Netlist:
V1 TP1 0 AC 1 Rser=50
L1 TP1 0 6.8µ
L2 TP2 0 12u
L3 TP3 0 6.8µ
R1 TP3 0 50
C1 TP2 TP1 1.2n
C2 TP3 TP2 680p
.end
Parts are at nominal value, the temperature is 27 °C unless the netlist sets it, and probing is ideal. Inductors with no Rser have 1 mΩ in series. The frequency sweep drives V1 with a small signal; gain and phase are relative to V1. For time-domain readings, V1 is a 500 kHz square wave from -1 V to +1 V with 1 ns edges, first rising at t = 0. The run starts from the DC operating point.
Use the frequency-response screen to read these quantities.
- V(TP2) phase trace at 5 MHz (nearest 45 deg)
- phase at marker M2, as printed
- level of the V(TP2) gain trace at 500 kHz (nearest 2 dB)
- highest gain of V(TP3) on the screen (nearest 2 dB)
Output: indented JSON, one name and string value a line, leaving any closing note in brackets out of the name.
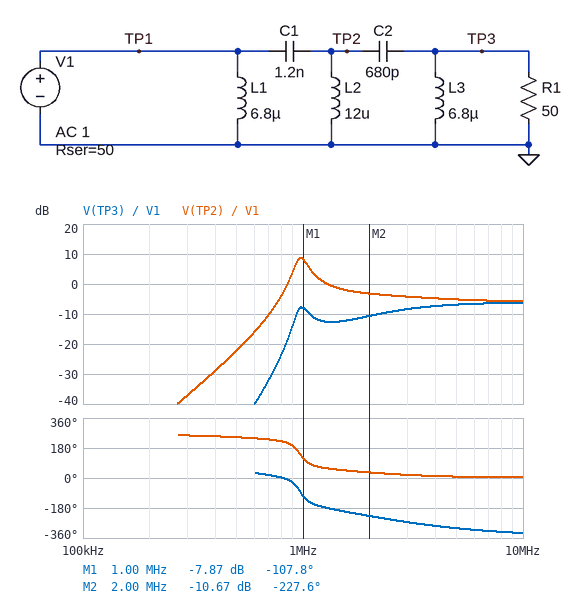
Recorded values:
{
  "V(TP2) phase trace at 5 MHz": "0 deg",
  "phase at marker M2, as printed": "-227.6 deg",
  "level of the V(TP2) gain trace at 500 kHz": "-22 dB",
  "highest gain of V(TP3) on the screen": "-6 dB"
}
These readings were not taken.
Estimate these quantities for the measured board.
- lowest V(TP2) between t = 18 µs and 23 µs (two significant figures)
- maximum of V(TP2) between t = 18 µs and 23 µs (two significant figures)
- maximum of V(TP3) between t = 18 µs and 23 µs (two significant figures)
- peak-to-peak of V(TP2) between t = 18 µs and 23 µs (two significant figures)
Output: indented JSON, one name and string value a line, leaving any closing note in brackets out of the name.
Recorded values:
{
  "lowest V(TP2) between t = 18 µs and 23 µs": "-810 mV",
  "maximum of V(TP2) between t = 18 µs and 23 µs": "810 mV",
  "maximum of V(TP3) between t = 18 µs and 23 µs": "1.0 V",
  "peak-to-peak of V(TP2) between t = 18 µs and 23 µs": "1.6 V"
}
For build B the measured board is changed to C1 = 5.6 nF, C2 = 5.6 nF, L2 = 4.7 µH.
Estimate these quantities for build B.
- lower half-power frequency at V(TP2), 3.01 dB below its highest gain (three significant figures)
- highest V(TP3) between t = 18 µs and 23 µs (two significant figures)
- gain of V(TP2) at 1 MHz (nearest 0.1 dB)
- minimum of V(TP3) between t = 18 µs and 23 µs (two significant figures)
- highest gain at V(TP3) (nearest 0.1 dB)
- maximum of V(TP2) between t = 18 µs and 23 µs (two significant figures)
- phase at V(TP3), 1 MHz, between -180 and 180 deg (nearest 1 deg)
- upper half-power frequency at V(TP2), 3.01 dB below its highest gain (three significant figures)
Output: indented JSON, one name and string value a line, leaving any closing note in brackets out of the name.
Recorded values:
{
  "lower half-power frequency at V(TP2), 3.01 dB below its highest gain": "508 kHz",
  "highest V(TP3) between t = 18 µs and 23 µs": "980 mV",
  "gain of V(TP2) at 1 MHz": "-9.8 dB",
  "minimum of V(TP3) between t = 18 µs and 23 µs": "-980 mV",
  "highest gain at V(TP3)": "-6.0 dB",
  "maximum of V(TP2) between t = 18 µs and 23 µs": "730 mV",
  "phase at V(TP3), 1 MHz, between -180 and 180 deg": "130 deg",
  "upper half-power frequency at V(TP2), 3.01 dB below its highest gain": "620 kHz"
}
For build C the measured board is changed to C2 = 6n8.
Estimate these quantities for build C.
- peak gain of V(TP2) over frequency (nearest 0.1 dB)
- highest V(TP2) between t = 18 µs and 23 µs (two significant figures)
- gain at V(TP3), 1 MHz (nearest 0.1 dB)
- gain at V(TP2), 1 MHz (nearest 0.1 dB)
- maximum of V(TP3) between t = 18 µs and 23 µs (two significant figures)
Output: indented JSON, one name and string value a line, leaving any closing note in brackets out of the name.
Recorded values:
{
  "peak gain of V(TP2) over frequency": "-6.0 dB",
  "highest V(TP2) between t = 18 µs and 23 µs": "1.1 V",
  "gain at V(TP3), 1 MHz": "-14.7 dB",
  "gain at V(TP2), 1 MHz": "-18.5 dB",
  "maximum of V(TP3) between t = 18 µs and 23 µs": "940 mV"
}
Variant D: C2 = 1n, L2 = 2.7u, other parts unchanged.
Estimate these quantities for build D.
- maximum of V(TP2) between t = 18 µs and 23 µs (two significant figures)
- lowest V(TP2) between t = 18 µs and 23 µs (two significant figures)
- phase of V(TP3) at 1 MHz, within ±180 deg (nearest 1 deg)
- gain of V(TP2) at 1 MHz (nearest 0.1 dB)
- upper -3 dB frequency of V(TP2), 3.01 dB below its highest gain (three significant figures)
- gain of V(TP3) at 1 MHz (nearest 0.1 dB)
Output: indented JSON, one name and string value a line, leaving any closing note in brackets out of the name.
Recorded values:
{
  "maximum of V(TP2) between t = 18 µs and 23 µs": "970 mV",
  "lowest V(TP2) between t = 18 µs and 23 µs": "-970 mV",
  "phase of V(TP3) at 1 MHz, within ±180 deg": "-15 deg",
  "gain of V(TP2) at 1 MHz": "-17.2 dB",
  "upper -3 dB frequency of V(TP2), 3.01 dB below its highest gain": "3.82 MHz",
  "gain of V(TP3) at 1 MHz": "-29.7 dB"
}
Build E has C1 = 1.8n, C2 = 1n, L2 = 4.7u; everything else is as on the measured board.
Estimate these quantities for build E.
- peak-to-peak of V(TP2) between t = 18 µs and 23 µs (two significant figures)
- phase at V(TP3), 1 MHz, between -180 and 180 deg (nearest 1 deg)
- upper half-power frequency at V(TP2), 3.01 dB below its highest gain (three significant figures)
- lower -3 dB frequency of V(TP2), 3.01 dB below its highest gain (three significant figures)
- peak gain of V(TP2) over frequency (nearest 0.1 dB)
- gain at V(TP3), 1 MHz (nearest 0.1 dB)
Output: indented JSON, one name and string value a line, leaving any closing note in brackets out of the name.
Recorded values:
{
  "peak-to-peak of V(TP2) between t = 18 µs and 23 µs": "2.1 V",
  "phase at V(TP3), 1 MHz, between -180 and 180 deg": "-43 deg",
  "upper half-power frequency at V(TP2), 3.01 dB below its highest gain": "1.61 MHz",
  "lower -3 dB frequency of V(TP2), 3.01 dB below its highest gain": "1.04 MHz",
  "peak gain of V(TP2) over frequency": "1.4 dB",
  "gain at V(TP3), 1 MHz": "-15.5 dB"
}
